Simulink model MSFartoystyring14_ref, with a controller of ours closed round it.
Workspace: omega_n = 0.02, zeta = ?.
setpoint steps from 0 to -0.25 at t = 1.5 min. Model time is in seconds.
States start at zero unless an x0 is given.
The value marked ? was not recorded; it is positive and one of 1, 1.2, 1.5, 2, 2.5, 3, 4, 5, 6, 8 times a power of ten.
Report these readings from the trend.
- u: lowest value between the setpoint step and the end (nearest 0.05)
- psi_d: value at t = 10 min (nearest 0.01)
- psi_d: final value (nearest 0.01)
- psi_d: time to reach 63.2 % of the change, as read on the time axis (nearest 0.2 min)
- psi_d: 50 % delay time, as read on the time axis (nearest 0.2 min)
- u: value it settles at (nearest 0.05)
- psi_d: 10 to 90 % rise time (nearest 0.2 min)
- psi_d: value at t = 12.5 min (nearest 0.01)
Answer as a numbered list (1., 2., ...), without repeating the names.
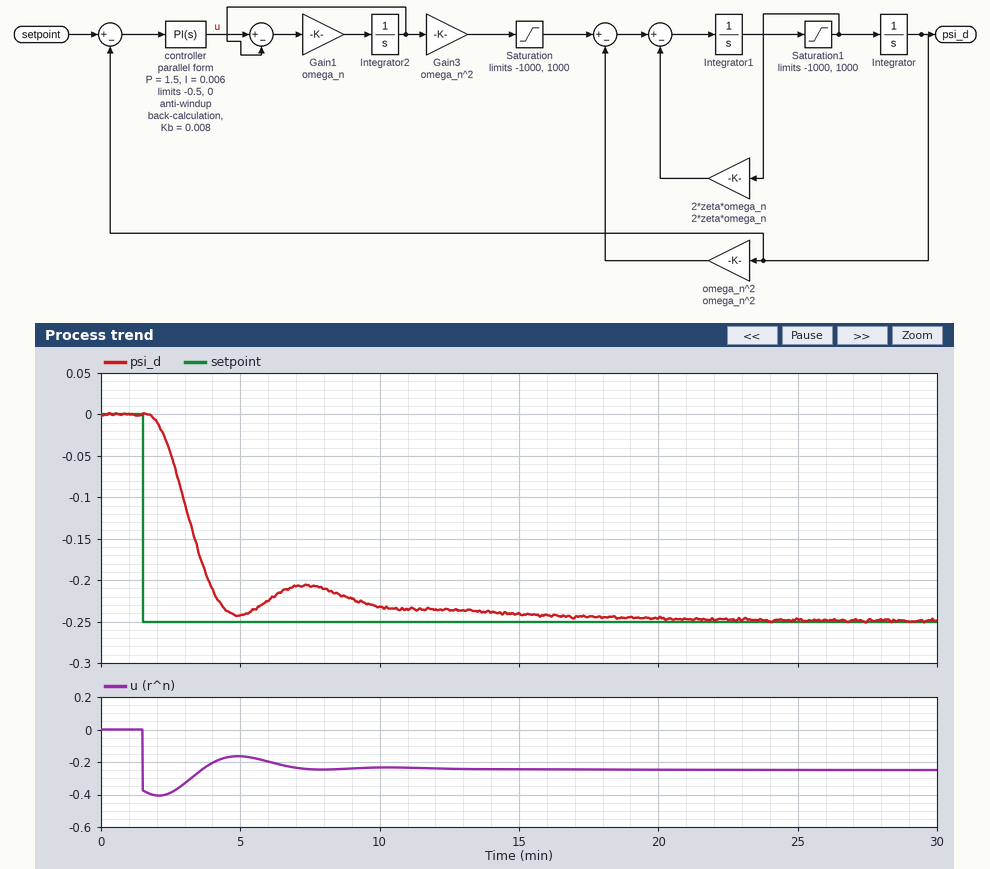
1. -0.40
2. -0.23
3. -0.25
4. 3.4 min
5. 3.2 min
6. -0.25
7. 2.0 min
8. -0.24
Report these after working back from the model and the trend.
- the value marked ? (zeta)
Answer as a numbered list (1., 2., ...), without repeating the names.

1. 1
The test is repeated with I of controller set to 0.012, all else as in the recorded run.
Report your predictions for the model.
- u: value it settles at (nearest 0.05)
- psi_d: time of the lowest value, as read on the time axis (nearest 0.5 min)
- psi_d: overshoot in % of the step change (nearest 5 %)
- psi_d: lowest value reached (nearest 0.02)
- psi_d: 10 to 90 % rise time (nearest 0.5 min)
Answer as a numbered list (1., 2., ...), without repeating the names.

1. -0.25
2. 5.0 min
3. 20 %
4. -0.30
5. 1.5 min
